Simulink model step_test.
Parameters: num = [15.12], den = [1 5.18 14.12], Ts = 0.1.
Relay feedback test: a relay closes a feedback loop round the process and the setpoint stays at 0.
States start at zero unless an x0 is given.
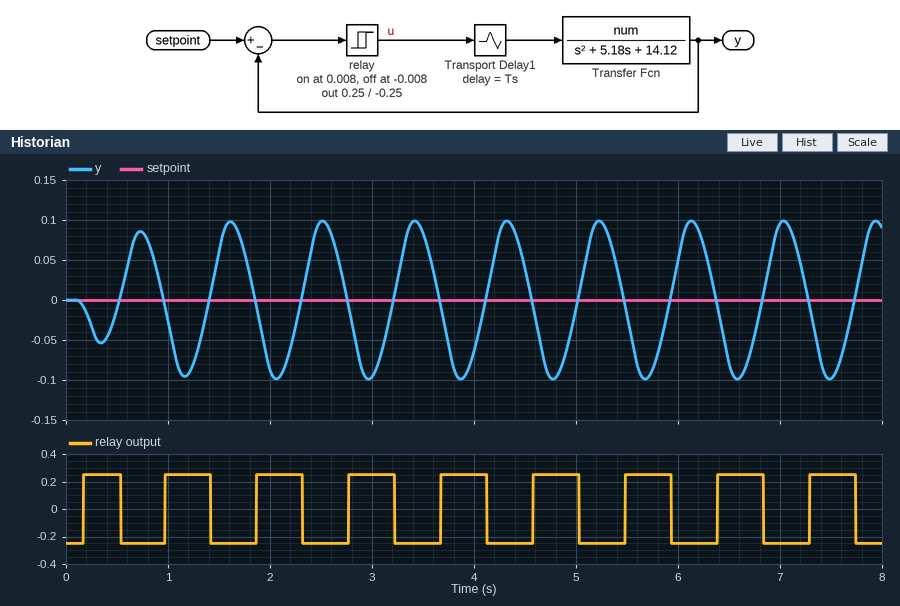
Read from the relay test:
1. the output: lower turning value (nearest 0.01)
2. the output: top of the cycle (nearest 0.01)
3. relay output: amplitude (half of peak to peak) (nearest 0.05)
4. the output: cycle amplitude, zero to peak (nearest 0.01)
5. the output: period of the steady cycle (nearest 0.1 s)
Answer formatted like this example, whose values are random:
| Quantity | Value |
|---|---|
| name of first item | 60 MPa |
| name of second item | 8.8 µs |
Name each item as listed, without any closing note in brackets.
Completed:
| Quantity | Value |
|---|---|
| the output: lower turning value | -0.10 |
| the output: top of the cycle | 0.10 |
| relay output: amplitude (half of peak to peak) | 0.25 |
| the output: cycle amplitude, zero to peak | 0.10 |
| the output: period of the steady cycle | 0.9 s |
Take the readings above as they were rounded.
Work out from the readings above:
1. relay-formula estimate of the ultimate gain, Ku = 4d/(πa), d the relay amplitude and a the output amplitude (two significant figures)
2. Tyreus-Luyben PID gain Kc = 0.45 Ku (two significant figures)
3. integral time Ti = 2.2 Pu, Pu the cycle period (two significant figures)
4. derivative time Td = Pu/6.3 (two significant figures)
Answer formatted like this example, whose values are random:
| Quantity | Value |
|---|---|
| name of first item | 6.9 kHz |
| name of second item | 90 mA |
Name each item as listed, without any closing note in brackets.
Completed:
| Quantity | Value |
|---|---|
| relay-formula estimate of the ultimate gain, Ku = 4d/(πa), d the relay amplitude and a the output amplitude | 3.2 |
| Tyreus-Luyben PID gain Kc = 0.45 Ku | 1.4 |
| integral time Ti = 2.2 Pu, Pu the cycle period | 2.0 s |
| derivative time Td = Pu/6.3 | 0.14 s |
